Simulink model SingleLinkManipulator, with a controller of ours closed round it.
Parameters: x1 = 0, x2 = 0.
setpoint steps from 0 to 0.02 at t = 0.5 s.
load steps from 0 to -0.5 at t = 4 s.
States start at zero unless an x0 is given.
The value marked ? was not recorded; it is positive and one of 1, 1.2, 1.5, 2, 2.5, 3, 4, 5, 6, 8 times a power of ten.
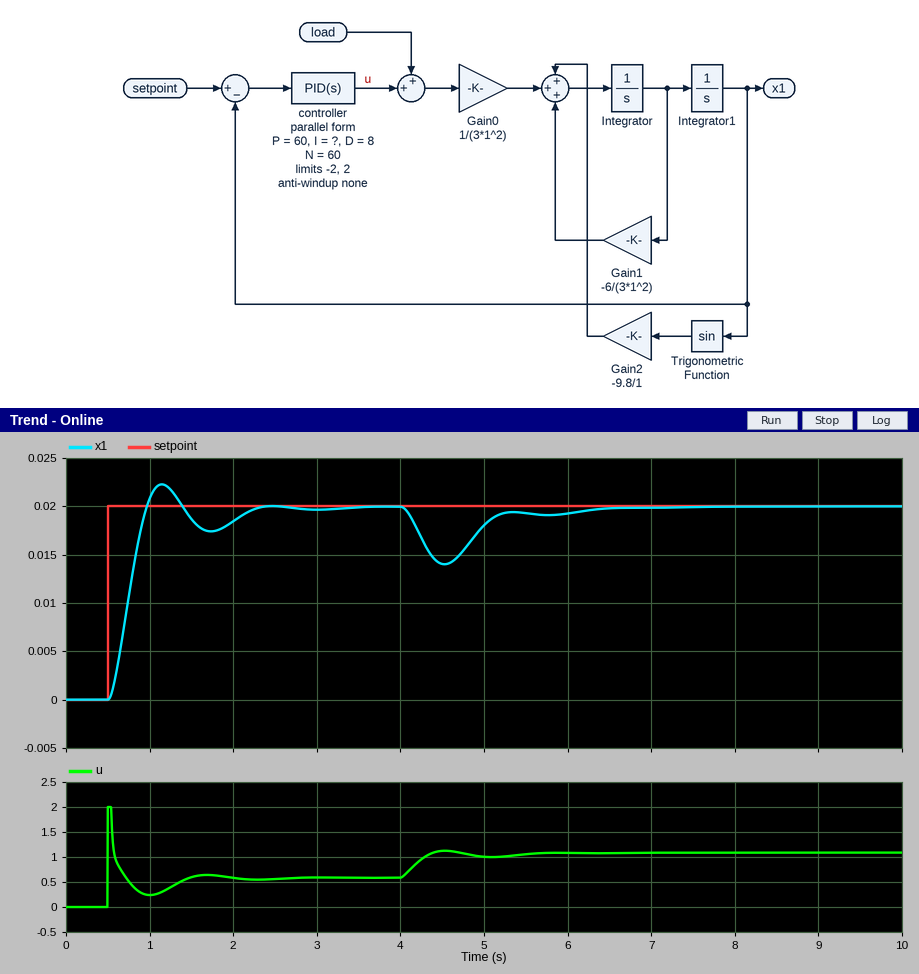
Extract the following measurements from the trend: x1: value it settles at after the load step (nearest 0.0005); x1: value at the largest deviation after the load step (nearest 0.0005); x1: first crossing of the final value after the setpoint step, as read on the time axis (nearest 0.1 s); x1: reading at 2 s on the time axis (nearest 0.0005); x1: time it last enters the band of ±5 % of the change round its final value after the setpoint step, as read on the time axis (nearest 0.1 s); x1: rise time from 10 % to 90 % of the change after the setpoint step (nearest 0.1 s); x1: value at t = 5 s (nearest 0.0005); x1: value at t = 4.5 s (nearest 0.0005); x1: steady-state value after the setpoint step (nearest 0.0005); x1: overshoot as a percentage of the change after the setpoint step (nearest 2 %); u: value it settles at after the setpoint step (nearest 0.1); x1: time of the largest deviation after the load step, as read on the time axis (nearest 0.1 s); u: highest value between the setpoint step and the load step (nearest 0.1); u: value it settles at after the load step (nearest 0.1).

0.0200
0.0140
1.0 s
0.0185
2.1 s
0.3 s
0.0180
0.0140
0.0200
12 %
0.6
4.5 s
2.0
1.1
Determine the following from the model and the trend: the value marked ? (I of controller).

100
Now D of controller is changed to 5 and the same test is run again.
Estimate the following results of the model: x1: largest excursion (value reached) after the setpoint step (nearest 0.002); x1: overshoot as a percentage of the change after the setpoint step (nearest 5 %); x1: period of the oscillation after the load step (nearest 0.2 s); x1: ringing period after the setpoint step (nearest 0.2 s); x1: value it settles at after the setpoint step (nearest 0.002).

0.024
20 %
1.2 s
1.2 s
0.020
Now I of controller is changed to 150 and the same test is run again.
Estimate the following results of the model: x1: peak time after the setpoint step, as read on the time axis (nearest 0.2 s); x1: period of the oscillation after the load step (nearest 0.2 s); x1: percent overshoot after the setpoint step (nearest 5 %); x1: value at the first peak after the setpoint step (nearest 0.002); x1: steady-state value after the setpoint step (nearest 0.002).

1.2 s
1.4 s
25 %
0.024
0.020
